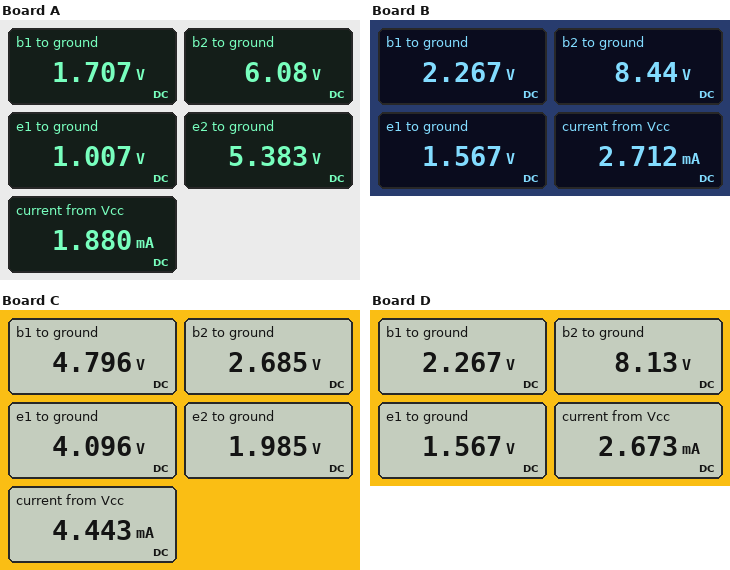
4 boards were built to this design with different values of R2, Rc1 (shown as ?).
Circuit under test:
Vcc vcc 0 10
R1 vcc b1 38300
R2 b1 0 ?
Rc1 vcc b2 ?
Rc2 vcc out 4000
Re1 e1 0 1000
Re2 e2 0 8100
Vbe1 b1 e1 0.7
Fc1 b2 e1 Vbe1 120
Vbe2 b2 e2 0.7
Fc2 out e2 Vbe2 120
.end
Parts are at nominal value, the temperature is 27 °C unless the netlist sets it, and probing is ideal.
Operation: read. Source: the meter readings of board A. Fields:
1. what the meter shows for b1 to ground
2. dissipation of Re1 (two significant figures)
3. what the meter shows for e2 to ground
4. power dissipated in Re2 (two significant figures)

1.707 V
1.0 mW
5.383 V
3.6 mW
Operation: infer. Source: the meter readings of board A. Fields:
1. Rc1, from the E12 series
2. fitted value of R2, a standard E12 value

3.9 kΩ
8.2 kΩ
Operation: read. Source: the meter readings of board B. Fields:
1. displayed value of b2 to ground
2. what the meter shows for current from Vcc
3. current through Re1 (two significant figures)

8.44 V
2.712 mA
1.6 mA
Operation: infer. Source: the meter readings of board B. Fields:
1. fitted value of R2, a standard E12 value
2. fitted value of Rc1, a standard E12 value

12 kΩ
1 kΩ
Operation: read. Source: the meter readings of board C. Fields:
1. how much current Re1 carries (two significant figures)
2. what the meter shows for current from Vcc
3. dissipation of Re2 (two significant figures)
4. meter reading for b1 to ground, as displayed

4.1 mA
4.443 mA
490 µW
4.796 V
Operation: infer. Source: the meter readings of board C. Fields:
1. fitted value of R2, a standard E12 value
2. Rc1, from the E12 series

47 kΩ
1.8 kΩ
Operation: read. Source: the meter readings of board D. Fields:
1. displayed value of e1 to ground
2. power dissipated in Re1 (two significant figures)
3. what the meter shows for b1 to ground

1.567 V
2.5 mW
2.267 V
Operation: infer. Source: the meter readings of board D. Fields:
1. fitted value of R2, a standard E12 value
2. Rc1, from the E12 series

12 kΩ
1.2 kΩ
